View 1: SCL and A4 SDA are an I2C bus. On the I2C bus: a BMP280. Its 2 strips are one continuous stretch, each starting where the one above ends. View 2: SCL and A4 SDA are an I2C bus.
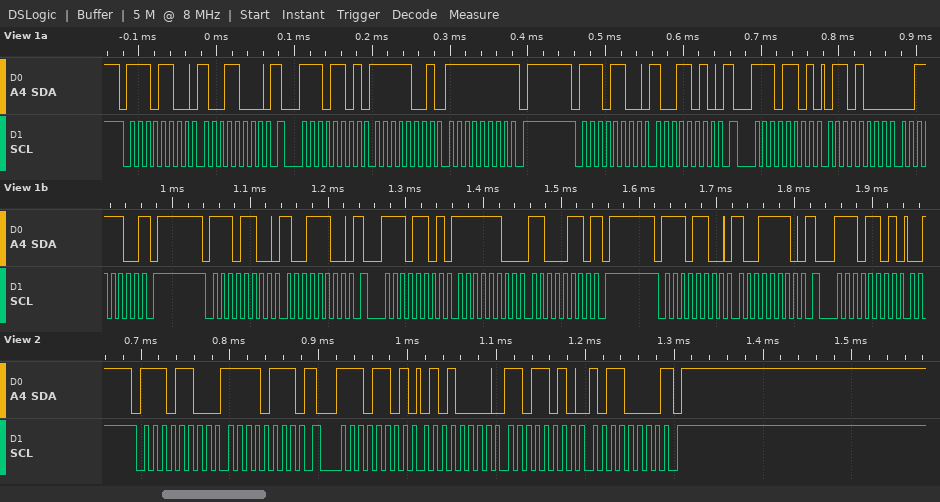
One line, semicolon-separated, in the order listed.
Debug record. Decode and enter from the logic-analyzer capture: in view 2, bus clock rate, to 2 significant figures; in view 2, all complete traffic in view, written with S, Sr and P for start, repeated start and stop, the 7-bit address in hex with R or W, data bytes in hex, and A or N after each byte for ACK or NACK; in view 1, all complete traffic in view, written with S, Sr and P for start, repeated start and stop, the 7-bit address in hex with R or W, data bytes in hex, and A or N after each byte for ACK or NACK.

100 kHz; S 76W A F7 A Sr 76R A 50 A DA A B0 N P; S 76W A 98 A Sr 76R A F9 A FF N P S 76W A 9A A Sr 76R A 68 A 3C N P S 76W A 9C A Sr 76R A FC A C6 N P S 76W A 9E A Sr 76R A
